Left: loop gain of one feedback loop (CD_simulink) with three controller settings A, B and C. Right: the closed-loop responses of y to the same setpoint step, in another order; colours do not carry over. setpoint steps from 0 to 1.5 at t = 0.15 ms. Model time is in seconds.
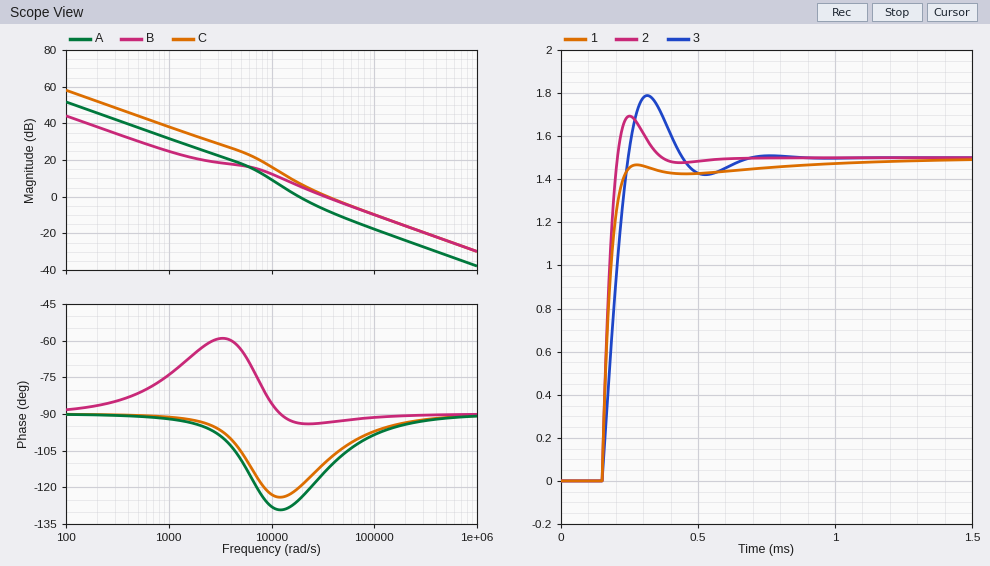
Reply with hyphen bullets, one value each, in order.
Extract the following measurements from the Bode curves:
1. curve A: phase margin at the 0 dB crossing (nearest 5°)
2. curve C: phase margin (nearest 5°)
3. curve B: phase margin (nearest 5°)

- 55°
- 70°
- 85°
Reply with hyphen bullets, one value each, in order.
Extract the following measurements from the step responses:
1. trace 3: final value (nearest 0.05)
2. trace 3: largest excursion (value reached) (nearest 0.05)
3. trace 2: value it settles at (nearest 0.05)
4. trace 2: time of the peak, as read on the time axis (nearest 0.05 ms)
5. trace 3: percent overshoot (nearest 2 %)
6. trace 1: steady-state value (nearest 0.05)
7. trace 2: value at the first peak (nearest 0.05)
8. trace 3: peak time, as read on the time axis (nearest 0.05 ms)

- 1.50
- 1.80
- 1.50
- 0.25 ms
- 20 %
- 1.50
- 1.70
- 0.30 ms
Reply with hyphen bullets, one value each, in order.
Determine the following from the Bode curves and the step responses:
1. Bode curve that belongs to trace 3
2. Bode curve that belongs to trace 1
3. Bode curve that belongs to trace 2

- A
- B
- C
